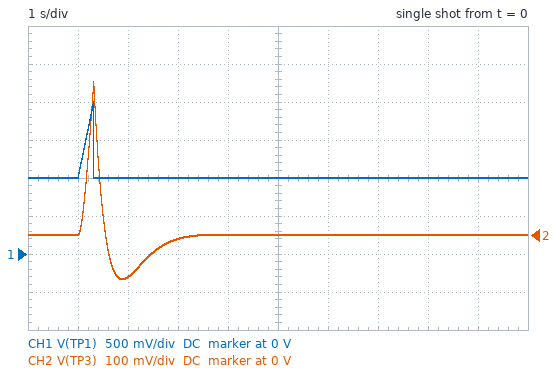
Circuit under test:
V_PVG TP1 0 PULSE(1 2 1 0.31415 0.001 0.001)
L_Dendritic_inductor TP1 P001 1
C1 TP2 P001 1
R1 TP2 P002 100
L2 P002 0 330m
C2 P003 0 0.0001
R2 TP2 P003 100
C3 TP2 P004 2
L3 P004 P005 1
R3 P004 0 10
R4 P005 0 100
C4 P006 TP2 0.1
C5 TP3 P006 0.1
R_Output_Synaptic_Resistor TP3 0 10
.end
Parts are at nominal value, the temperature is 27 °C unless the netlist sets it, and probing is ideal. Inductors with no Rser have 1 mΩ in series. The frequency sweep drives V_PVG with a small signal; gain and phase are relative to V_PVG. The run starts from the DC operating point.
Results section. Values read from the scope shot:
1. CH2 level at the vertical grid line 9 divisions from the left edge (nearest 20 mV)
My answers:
0 V
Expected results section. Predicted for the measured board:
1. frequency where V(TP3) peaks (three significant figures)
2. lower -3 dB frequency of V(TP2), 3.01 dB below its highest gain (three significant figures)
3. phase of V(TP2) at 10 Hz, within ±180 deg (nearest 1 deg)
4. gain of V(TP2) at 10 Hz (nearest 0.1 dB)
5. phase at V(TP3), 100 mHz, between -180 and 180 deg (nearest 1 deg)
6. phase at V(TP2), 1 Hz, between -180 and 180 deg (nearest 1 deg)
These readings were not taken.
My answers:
489 mHz
28.8 mHz
-86 deg
-22.8 dB
79 deg
-58 deg
